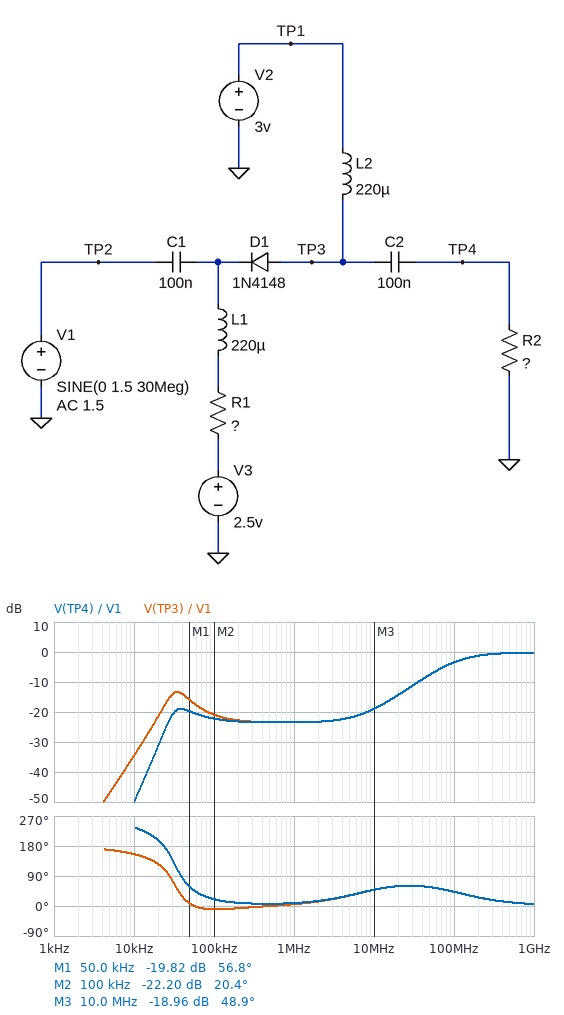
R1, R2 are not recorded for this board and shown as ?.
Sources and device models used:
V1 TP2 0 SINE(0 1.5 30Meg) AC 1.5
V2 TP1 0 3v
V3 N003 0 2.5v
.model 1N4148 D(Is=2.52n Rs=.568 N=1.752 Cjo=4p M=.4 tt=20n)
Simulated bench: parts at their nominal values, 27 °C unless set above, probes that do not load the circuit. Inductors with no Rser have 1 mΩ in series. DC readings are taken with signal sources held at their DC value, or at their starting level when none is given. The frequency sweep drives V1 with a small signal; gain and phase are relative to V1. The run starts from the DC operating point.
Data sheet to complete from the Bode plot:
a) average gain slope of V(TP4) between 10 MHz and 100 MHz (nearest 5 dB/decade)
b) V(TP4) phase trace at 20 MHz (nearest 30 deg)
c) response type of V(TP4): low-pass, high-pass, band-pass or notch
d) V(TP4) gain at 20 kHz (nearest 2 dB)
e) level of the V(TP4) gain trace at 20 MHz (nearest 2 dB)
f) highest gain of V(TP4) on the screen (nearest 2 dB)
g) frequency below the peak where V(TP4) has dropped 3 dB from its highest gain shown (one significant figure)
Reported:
15 dB/decade
60 deg
high-pass
-32 dB
-14 dB
0 dB
100 MHz
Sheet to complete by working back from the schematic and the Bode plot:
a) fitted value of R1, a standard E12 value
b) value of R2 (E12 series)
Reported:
100 Ω
27 Ω
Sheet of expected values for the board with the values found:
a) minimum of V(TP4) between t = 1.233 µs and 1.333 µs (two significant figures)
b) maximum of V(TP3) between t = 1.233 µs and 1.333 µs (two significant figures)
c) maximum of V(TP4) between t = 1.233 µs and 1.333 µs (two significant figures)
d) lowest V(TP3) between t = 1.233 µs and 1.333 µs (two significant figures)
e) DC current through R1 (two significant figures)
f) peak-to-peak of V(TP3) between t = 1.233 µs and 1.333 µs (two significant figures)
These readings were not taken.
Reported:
-1.1 V
4.4 V
1.5 V
1.8 V
120 µA
2.6 V
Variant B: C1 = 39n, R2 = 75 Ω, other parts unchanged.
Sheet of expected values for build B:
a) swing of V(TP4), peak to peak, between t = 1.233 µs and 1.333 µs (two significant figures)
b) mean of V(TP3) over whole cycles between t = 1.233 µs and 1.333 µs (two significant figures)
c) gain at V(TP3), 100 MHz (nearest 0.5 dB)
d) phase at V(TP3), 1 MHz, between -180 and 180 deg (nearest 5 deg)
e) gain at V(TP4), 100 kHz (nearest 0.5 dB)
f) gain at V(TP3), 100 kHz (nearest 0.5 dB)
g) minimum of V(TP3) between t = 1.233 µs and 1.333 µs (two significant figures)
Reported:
2.8 V
2.9 V
-1.0 dB
10 deg
-14.5 dB
-14.0 dB
1.7 V
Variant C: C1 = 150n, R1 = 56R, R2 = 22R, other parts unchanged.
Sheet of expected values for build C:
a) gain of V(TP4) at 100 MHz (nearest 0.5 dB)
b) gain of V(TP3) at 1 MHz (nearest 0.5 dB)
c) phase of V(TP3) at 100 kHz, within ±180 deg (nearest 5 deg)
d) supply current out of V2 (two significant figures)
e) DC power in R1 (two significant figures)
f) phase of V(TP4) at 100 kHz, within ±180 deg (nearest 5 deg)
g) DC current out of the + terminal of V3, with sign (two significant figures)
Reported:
-4.0 dB
-24.5 dB
-20 deg
130 µA
980 nW
15 deg
-130 µA
